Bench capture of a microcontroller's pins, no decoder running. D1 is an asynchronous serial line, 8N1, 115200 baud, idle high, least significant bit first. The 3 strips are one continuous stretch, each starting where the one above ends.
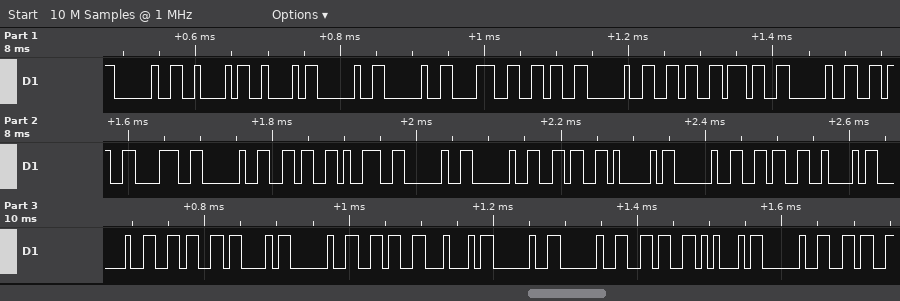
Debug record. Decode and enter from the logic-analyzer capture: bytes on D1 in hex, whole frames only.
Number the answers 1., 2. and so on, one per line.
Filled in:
1. 20 42 42 20 20 38 36 20 36 37 20 36 38 20 36 39 20 20 36 41 20 36 42 20 36 43 20 36 44 20 20 36 45 20 36
